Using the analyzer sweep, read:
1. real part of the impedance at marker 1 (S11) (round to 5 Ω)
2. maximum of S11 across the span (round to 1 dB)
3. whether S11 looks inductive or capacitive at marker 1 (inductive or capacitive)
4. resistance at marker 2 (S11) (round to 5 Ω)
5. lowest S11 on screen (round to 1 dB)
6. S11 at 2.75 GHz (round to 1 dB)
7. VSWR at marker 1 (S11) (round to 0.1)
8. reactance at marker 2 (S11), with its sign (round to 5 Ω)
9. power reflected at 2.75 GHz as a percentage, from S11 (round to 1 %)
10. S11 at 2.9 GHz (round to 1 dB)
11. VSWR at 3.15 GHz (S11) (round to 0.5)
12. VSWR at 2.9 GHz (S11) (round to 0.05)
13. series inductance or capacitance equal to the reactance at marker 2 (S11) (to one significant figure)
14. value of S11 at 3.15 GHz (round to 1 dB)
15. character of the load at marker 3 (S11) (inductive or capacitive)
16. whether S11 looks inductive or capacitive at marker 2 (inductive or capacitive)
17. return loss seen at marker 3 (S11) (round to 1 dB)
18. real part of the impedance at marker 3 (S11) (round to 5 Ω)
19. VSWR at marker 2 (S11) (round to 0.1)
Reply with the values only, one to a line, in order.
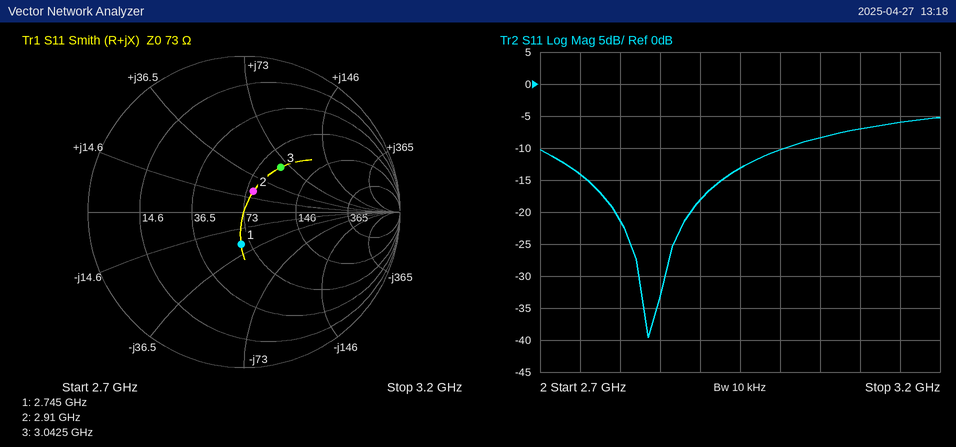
65 Ω
-5 dB
capacitive
80 Ω
-40 dB
-14 dB
1.5
+20 Ω
4 %
-18 dB
3.0
1.30
1 nH
-6 dB
inductive
inductive
9 dB
95 Ω
1.3
